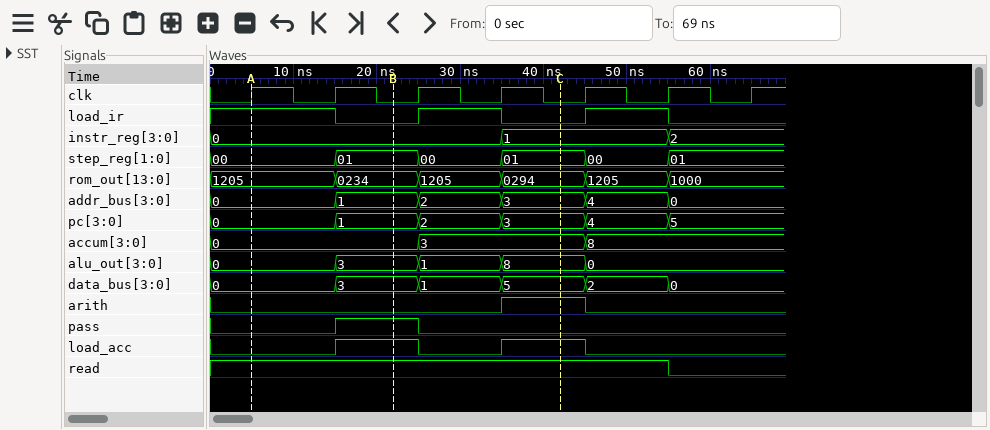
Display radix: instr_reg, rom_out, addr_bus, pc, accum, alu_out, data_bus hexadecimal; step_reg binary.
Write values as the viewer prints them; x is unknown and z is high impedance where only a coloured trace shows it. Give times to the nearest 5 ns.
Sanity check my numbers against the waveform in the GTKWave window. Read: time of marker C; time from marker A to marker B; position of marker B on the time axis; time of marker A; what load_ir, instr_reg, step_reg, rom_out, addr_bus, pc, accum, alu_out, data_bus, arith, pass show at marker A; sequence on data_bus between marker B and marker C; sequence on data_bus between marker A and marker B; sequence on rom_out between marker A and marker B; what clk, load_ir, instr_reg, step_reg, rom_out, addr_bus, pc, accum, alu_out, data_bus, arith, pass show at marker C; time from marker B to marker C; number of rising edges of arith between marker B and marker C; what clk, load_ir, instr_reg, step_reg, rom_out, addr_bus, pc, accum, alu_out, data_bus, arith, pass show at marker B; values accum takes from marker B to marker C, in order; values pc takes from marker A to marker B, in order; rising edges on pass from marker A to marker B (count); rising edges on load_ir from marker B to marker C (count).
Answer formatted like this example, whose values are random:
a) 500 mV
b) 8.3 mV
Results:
a) 40 ns
b) 15 ns
c) 20 ns
d) 5 ns
e) load_ir=1, instr_reg=0, step_reg=00, rom_out=1205, addr_bus=0, pc=0, accum=0, alu_out=0, data_bus=0, arith=0, pass=0
f) 3, 1, 5
g) 0, 3
h) 1205, 0234
i) clk=0, load_ir=0, instr_reg=1, step_reg=01, rom_out=0294, addr_bus=3, pc=3, accum=3, alu_out=8, data_bus=5, arith=1, pass=0
j) 20 ns
k) 1
l) clk=0, load_ir=0, instr_reg=0, step_reg=01, rom_out=0234, addr_bus=1, pc=1, accum=0, alu_out=3, data_bus=3, arith=0, pass=1
m) 0, 3
n) 0, 1
o) 1
p) 1
